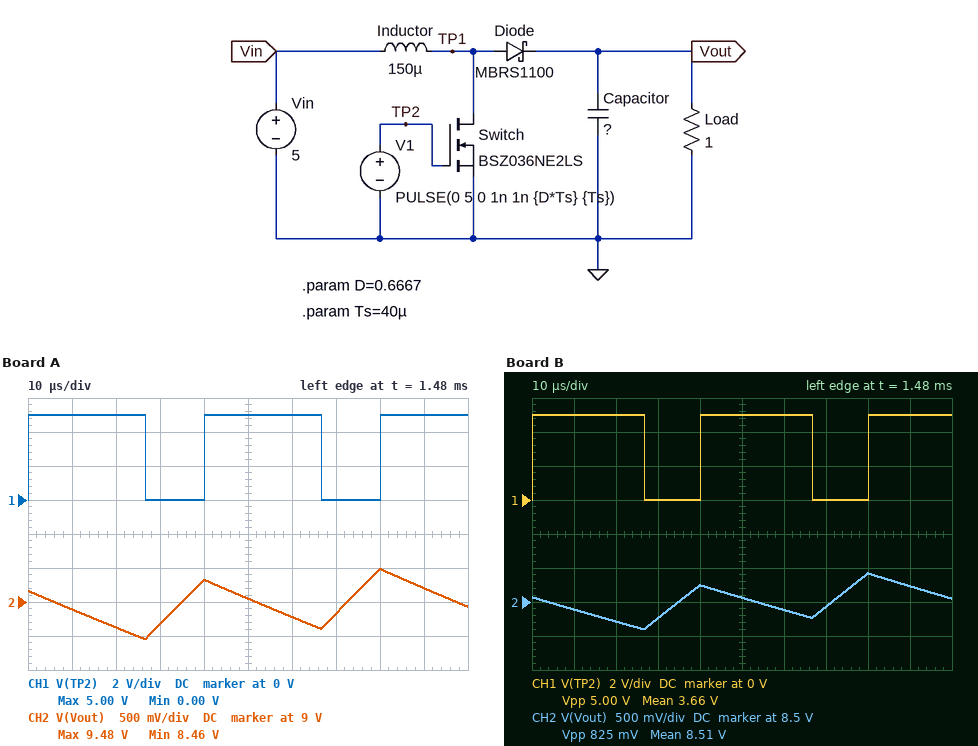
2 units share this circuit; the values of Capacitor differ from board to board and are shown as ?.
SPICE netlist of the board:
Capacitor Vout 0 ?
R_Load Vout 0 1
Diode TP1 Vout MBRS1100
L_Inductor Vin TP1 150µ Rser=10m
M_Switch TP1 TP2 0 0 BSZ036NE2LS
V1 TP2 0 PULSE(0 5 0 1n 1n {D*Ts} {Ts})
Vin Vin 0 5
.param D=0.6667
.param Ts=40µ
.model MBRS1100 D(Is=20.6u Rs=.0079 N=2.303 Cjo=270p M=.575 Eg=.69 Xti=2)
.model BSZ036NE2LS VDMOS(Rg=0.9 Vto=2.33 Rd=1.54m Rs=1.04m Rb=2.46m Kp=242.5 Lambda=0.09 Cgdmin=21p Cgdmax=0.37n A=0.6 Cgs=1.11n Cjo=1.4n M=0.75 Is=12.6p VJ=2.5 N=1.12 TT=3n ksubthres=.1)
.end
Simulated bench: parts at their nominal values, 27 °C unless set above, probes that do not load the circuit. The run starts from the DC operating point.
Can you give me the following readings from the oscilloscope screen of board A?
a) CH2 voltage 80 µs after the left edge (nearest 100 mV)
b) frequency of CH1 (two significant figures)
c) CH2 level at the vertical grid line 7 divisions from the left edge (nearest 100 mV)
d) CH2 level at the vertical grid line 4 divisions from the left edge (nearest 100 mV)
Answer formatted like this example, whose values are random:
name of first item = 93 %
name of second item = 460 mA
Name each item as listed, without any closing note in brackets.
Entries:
CH2 voltage 80 µs after the left edge = 9.5 V
frequency of CH1 = 25 kHz
CH2 level at the vertical grid line 7 divisions from the left edge = 8.8 V
CH2 level at the vertical grid line 4 divisions from the left edge = 9.3 V
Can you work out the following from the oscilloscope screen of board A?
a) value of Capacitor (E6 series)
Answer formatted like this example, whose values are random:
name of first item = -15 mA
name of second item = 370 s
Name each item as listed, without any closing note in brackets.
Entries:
value of Capacitor = 330 µF
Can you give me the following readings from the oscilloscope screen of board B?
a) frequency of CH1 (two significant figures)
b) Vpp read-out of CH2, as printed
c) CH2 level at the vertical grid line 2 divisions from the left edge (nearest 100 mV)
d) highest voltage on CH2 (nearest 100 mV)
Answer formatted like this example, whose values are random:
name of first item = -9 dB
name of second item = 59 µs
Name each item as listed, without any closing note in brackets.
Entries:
frequency of CH1 = 25 kHz
Vpp read-out of CH2, as printed = 825 mV
CH2 level at the vertical grid line 2 divisions from the left edge = 8.2 V
highest voltage on CH2 = 8.9 V
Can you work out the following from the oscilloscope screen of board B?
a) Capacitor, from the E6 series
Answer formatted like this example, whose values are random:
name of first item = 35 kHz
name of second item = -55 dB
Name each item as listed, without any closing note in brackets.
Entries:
Capacitor, from the E6 series = 470 µF
